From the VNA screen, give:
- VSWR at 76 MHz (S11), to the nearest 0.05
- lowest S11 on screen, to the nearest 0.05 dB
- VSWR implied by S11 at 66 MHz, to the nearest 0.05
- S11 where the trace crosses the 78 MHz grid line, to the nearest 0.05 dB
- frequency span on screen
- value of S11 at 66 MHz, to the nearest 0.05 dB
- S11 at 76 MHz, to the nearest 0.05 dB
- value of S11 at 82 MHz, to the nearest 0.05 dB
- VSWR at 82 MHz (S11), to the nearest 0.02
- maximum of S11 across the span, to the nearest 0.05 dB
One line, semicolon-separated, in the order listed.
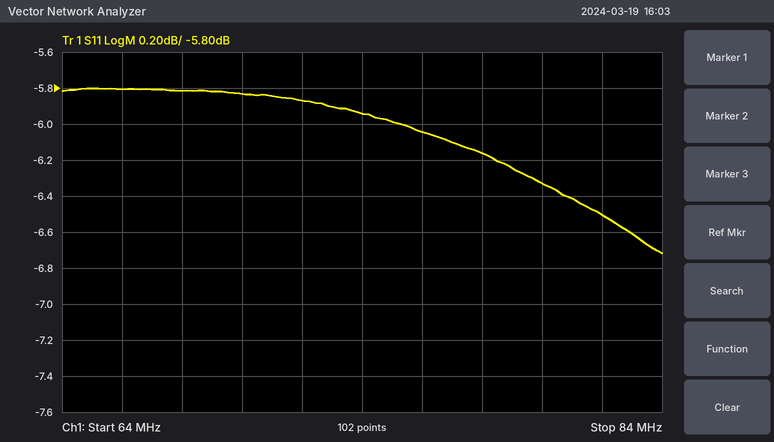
3.00; -6.70 dB; 3.10; -6.15 dB; 20 MHz; -5.80 dB; -6.05 dB; -6.50 dB; 2.80; -5.80 dB
